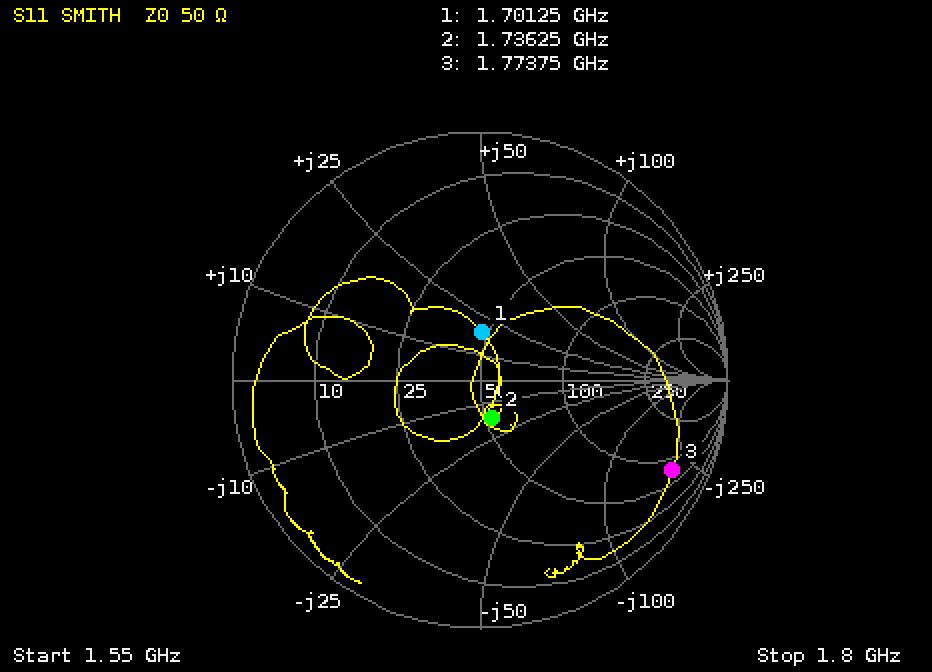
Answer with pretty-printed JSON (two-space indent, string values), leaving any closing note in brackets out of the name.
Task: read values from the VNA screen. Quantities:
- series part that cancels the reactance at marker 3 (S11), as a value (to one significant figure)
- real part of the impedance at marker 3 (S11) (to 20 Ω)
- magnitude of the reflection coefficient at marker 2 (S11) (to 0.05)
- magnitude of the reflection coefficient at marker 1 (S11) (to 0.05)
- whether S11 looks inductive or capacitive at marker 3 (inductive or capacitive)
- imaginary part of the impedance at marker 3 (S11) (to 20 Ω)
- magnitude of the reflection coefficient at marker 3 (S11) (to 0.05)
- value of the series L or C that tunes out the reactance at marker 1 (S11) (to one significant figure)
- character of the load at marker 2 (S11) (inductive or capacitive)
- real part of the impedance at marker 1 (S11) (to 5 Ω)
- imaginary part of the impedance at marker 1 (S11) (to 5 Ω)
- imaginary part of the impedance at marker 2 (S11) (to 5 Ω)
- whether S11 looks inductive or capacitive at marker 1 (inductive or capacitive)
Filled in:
{
  "series part that cancels the reactance at marker 3 (S11), as a value": "20 nH",
  "real part of the impedance at marker 3 (S11)": "80 Ω",
  "magnitude of the reflection coefficient at marker 2 (S11)": "0.15",
  "magnitude of the reflection coefficient at marker 1 (S11)": "0.20",
  "whether S11 looks inductive or capacitive at marker 3": "capacitive",
  "imaginary part of the impedance at marker 3 (S11)": "-200 Ω",
  "magnitude of the reflection coefficient at marker 3 (S11)": "0.85",
  "value of the series L or C that tunes out the reactance at marker 1 (S11)": "5 pF",
  "character of the load at marker 2 (S11)": "capacitive",
  "real part of the impedance at marker 1 (S11)": "45 Ω",
  "imaginary part of the impedance at marker 1 (S11)": "+20 Ω",
  "imaginary part of the impedance at marker 2 (S11)": "-15 Ω",
  "whether S11 looks inductive or capacitive at marker 1": "inductive"
}
